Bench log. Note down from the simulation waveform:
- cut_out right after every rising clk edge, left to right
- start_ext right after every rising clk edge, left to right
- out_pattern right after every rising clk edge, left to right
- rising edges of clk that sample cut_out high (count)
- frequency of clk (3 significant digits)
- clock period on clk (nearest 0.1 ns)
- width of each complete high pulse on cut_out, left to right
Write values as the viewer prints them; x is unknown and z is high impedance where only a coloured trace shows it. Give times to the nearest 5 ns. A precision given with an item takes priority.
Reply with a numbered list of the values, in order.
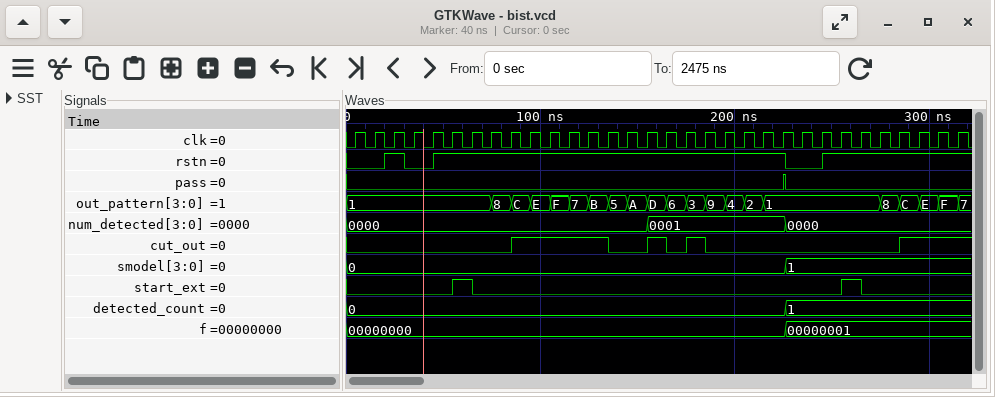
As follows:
1. 0 0 0 0 0 0 0 0 1 1 1 1 1 0 0 1 0 1 0 0 0 0 0 0 0 0 0 0 1 1 1 1
2. 0 0 0 0 0 1 0 0 0 0 0 0 0 0 0 0 0 0 0 0 0 0 0 0 0 1 0 0 0 0 0 0
3. 1, 1, 1, 1, 1, 1, 1, 8, C, E, F, 7, B, 5, A, D, 6, 3, 9, 4, 2, 1, 1, 1, 1, 1, 1, 8, C, E, F, 7
4. 10
5. 100 MHz
6. 10 ns
7. 50 ns, 10 ns, 10 ns
